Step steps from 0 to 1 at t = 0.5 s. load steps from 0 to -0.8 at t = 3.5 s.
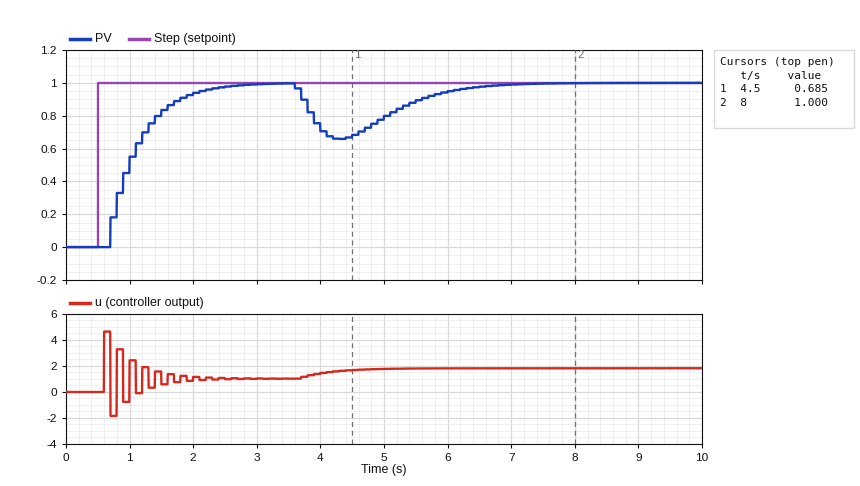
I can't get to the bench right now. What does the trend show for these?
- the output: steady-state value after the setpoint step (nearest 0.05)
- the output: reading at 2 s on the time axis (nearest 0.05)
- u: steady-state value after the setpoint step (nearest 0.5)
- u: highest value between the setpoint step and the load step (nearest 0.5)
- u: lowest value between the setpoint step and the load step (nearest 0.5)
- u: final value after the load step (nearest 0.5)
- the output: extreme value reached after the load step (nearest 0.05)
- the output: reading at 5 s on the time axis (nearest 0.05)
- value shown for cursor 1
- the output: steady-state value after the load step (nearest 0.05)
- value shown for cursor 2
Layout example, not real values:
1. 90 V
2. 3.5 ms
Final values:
1. 1.00
2. 0.95
3. 1.0
4. 4.5
5. -2.0
6. 2.0
7. 0.65
8. 0.80
9. 0.685
10. 1.00
11. 1.000
